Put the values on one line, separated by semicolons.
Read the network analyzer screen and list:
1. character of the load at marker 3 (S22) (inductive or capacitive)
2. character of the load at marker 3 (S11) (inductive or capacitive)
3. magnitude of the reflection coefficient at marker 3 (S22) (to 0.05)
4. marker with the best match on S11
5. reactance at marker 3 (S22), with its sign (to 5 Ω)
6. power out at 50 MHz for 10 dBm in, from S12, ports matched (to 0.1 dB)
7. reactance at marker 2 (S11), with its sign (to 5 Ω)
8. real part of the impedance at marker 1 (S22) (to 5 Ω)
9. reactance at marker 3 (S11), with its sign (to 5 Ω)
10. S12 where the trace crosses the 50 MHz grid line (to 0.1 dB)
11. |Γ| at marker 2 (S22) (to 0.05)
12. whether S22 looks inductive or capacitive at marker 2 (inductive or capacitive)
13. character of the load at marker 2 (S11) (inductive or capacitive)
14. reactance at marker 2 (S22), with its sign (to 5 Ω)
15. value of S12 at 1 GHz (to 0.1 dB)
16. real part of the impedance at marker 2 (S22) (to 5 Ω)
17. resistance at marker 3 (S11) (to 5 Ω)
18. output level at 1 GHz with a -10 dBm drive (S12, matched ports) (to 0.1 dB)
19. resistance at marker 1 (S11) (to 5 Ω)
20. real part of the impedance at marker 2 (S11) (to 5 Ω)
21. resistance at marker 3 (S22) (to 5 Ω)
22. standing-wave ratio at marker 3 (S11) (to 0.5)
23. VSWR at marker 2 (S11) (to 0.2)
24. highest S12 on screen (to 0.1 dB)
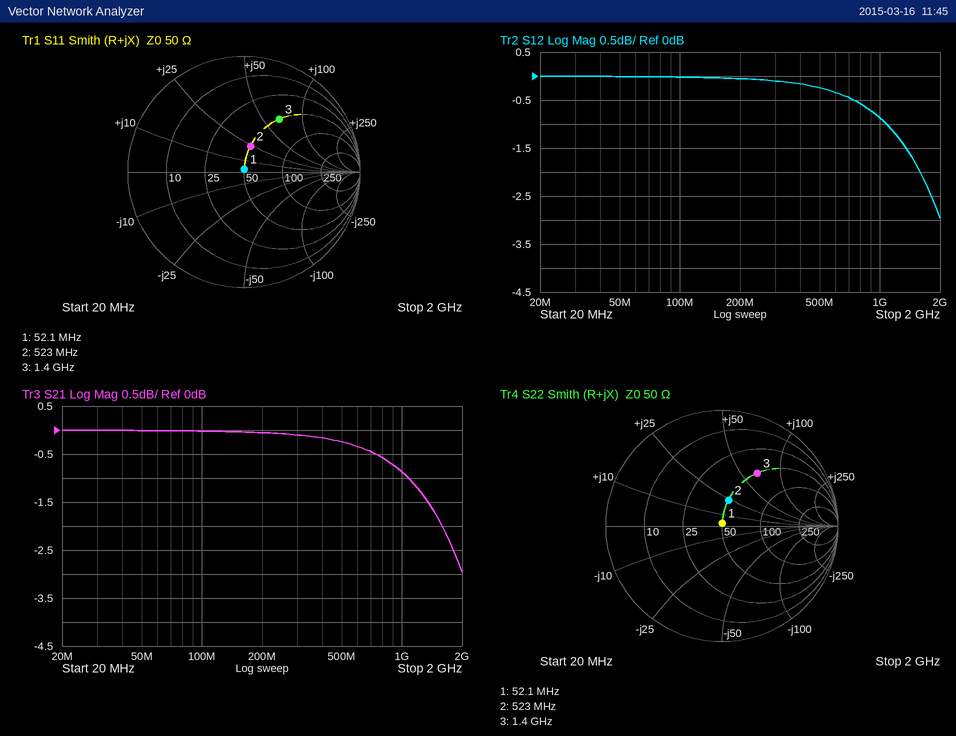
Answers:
inductive; inductive; 0.55; marker 1; +65 Ω; 10.0 dBm; +25 Ω; 50 Ω; +65 Ω; 0.0 dB; 0.25; inductive; inductive; +25 Ω; -0.9 dB; 50 Ω; 50 Ω; -10.9 dBm; 50 Ω; 50 Ω; 50 Ω; 3.5; 1.6; 0.0 dB
